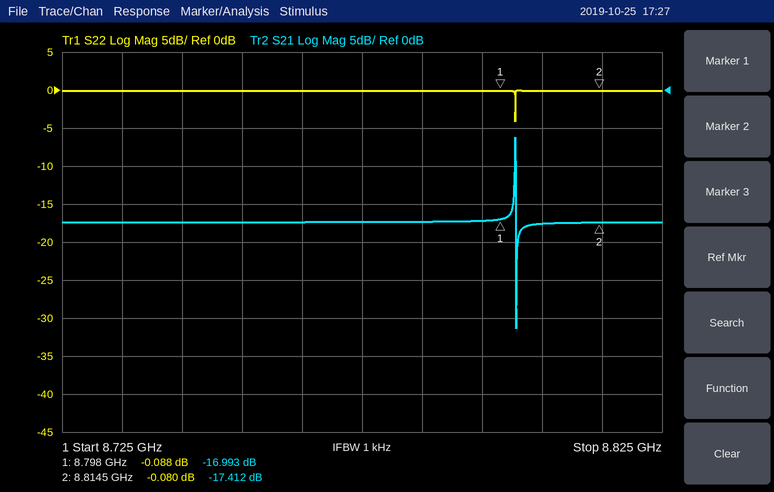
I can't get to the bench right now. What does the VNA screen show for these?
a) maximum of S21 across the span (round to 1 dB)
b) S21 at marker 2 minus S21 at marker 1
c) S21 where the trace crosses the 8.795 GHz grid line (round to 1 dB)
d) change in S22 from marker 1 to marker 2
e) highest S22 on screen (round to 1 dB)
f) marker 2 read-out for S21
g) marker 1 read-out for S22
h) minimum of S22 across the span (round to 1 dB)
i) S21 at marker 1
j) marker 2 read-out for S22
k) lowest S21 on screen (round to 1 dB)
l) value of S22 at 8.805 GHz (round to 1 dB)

-6 dB
-0.419 dB
-17 dB
0.008 dB
0 dB
-17.412 dB
-0.088 dB
-4 dB
-16.993 dB
-0.080 dB
-31 dB
0 dB
